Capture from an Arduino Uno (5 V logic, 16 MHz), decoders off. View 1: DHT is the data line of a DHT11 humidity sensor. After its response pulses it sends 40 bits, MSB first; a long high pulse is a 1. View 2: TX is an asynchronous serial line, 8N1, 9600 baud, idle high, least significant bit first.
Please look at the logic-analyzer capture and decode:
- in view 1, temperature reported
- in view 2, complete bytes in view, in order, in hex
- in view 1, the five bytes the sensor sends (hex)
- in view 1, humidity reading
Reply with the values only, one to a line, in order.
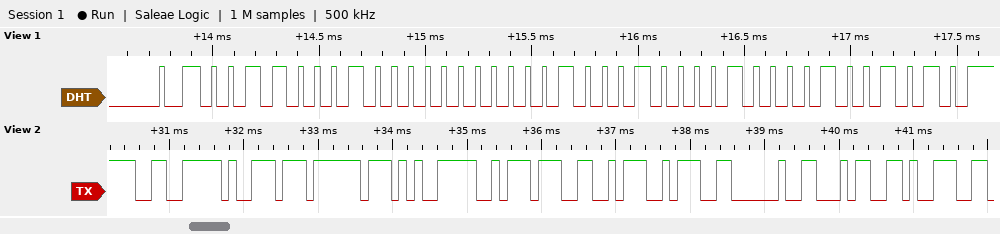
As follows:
17.8 °C
0xE6 0xB9 0xBF 0xE5 0xBA 0xA6 0x3A 0x20 0x34 0x39
31 00 11 08 4A
49 %
